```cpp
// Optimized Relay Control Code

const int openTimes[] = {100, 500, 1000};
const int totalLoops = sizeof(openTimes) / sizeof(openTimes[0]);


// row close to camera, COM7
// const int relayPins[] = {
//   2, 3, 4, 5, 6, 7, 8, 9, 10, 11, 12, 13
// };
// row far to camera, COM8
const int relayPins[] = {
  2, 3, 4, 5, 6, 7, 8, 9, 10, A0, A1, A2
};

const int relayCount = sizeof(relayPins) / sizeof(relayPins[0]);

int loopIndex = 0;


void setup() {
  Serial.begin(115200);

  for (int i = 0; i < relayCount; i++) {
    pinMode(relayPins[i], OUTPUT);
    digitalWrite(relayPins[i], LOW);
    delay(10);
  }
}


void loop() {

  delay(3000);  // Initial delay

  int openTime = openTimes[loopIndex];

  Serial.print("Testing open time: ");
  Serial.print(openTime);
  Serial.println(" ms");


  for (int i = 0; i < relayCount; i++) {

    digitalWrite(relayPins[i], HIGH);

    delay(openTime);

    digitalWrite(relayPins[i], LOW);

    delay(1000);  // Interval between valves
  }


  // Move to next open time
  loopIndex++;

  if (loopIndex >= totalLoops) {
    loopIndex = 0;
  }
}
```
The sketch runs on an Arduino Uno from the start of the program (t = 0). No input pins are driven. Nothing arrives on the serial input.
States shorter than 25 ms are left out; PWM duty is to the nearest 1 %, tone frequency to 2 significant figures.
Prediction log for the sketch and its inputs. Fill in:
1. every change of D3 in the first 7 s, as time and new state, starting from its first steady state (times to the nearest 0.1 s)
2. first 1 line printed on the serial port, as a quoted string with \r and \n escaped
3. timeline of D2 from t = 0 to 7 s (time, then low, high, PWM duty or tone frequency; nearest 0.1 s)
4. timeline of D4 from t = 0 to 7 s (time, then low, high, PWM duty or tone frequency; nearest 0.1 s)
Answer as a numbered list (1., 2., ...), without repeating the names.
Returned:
1. 0 s low; 4.2 s high; 4.3 s low
2. "Testing open time: 100 ms\r\n"
3. 0 s low; 3.1 s high; 3.2 s low
4. 0 s low; 5.3 s high; 5.4 s low
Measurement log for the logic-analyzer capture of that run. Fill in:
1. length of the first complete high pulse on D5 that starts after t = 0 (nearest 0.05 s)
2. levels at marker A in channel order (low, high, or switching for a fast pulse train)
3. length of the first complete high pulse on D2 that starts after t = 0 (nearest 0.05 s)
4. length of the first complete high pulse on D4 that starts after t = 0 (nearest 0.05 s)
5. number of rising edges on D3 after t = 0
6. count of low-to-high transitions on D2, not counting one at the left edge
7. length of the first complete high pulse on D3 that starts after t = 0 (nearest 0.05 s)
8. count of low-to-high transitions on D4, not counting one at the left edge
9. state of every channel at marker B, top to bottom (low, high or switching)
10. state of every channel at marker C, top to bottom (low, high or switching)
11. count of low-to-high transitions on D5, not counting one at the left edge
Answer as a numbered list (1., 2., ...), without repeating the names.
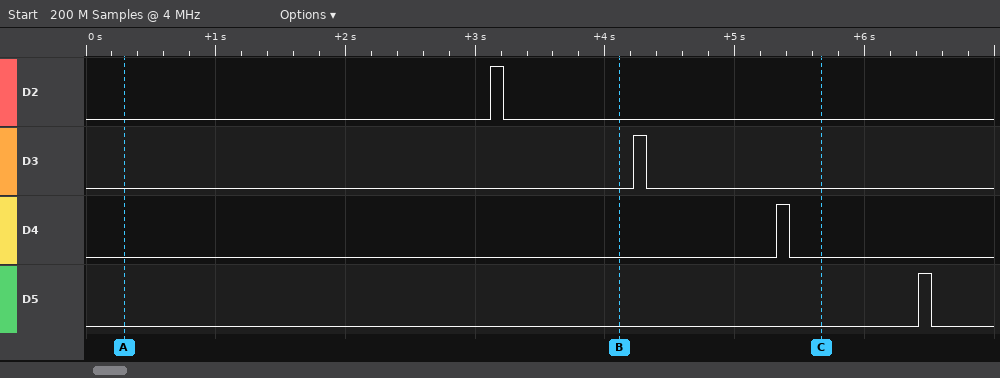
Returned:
1. 0.10 s
2. D2 low, D3 low, D4 low, D5 low
3. 0.10 s
4. 0.10 s
5. 1
6. 1
7. 0.10 s
8. 1
9. D2 low, D3 low, D4 low, D5 low
10. D2 low, D3 low, D4 low, D5 low
11. 1
